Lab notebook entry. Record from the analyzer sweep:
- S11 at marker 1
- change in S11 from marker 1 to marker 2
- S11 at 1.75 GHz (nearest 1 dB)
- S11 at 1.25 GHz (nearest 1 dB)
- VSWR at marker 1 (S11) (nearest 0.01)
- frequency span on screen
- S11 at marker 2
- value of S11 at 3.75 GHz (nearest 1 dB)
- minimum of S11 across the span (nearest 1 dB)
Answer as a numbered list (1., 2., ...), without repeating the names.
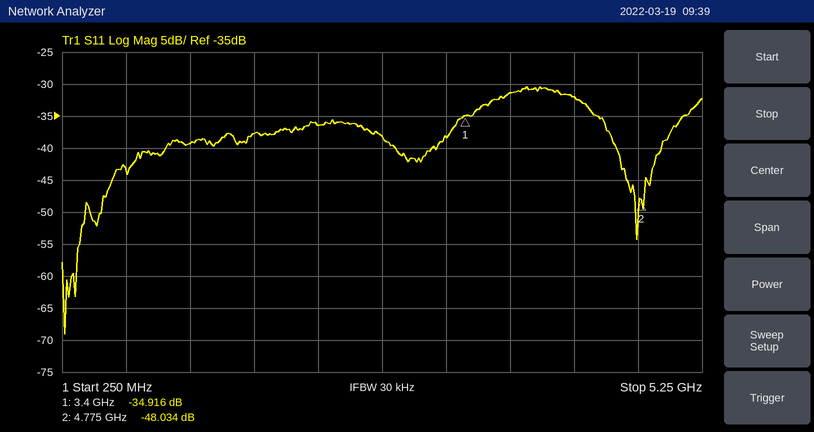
1. -34.916 dB
2. -13.118 dB
3. -38 dB
4. -39 dB
5. 1.04
6. 5 GHz
7. -48.034 dB
8. -31 dB
9. -69 dB
